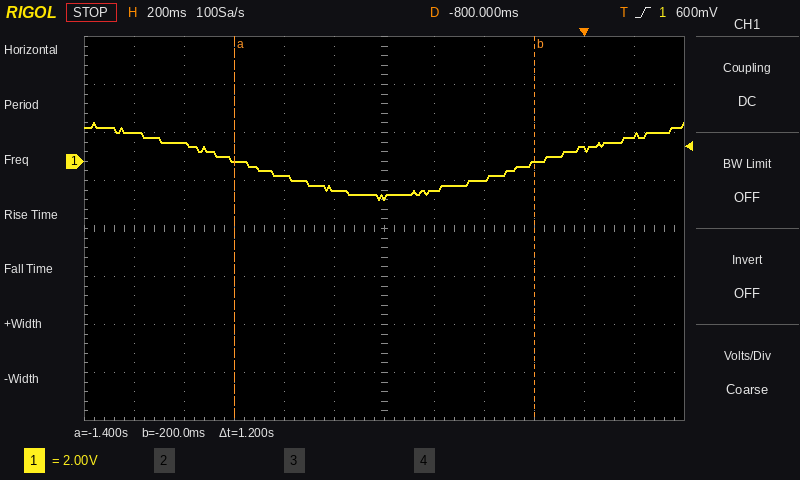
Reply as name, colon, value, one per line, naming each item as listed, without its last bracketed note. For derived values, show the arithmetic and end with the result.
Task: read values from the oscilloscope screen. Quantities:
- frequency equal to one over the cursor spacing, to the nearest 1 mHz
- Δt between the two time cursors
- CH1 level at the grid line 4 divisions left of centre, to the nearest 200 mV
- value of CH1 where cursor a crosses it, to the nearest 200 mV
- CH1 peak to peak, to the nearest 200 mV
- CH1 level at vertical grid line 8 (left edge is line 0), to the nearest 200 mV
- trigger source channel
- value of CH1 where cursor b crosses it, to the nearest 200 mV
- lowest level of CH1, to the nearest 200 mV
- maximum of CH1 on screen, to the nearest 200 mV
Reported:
frequency equal to one over the cursor spacing, to the nearest 1 mHz: 1 / 1.2 s ≈ 833 mHz
Δt between the two time cursors: 1.2 s
CH1 level at the grid line 4 divisions left of centre, to the nearest 200 mV: 800 mV
value of CH1 where cursor a crosses it, to the nearest 200 mV: 0.0 V
CH1 peak to peak, to the nearest 200 mV: 1.6 V − (-1.6 V) = 3.2 V
CH1 level at vertical grid line 8 (left edge is line 0), to the nearest 200 mV: -800 mV
trigger source channel: CH1
value of CH1 where cursor b crosses it, to the nearest 200 mV: 0.0 V
lowest level of CH1, to the nearest 200 mV: -1.6 V
maximum of CH1 on screen, to the nearest 200 mV: 1.6 V
